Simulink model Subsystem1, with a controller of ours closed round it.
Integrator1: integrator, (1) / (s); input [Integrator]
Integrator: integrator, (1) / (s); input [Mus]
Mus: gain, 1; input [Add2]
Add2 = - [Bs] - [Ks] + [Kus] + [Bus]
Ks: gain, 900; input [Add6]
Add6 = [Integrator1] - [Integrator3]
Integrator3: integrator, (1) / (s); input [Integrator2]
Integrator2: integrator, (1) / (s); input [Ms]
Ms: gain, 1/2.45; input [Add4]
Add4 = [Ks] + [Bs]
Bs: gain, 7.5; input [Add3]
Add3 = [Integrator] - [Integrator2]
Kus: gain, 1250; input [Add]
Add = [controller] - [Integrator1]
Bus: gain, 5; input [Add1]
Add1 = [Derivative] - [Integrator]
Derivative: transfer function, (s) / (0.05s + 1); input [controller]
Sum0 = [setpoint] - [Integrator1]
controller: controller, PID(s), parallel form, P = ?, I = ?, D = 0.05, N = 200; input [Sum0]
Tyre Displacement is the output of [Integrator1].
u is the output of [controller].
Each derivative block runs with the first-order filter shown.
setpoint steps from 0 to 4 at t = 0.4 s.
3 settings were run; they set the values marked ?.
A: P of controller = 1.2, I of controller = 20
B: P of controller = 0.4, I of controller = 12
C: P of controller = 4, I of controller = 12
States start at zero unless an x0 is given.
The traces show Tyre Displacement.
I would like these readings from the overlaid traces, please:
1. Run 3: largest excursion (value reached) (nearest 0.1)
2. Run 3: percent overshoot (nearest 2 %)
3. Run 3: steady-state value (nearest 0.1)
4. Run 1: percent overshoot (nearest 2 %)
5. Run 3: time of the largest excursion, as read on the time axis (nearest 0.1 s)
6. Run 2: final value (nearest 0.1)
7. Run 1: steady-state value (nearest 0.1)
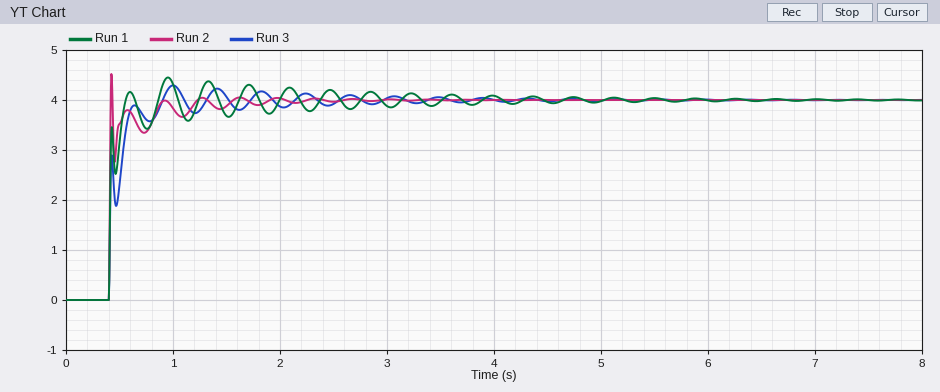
4.3
8 %
4.0
12 %
1.0 s
4.0
4.0
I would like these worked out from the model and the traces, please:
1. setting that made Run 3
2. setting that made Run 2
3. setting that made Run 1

B
C
A
